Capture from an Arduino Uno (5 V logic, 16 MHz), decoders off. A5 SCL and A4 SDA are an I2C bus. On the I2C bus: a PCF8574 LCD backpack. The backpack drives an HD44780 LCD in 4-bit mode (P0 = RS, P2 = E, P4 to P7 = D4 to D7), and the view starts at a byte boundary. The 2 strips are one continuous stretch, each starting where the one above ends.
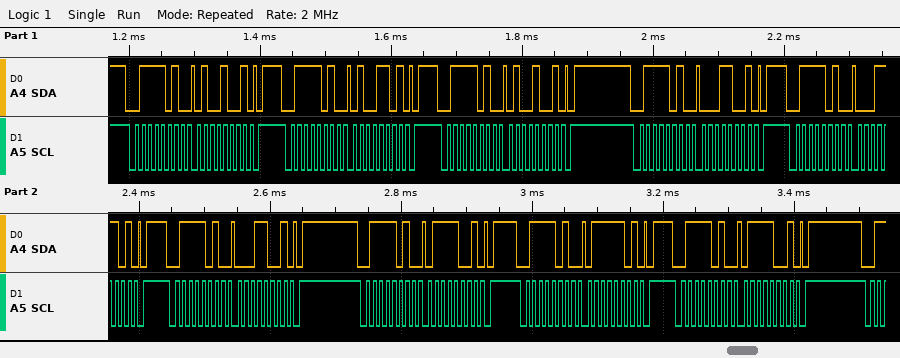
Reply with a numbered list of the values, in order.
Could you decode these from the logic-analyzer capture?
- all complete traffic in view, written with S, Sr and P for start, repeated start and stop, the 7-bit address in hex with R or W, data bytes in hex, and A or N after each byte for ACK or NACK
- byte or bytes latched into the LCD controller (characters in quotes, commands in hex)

1. S 3DW A 49 A P S 3DW A 4D A P S 3DW A 49 A P S 3DW A 19 A P S 3DW A 1D A P S 3DW A 19 A P S 3DW A 79 A P S 3DW A 7D A P S 3DW A 79 A P
2. 'A'
